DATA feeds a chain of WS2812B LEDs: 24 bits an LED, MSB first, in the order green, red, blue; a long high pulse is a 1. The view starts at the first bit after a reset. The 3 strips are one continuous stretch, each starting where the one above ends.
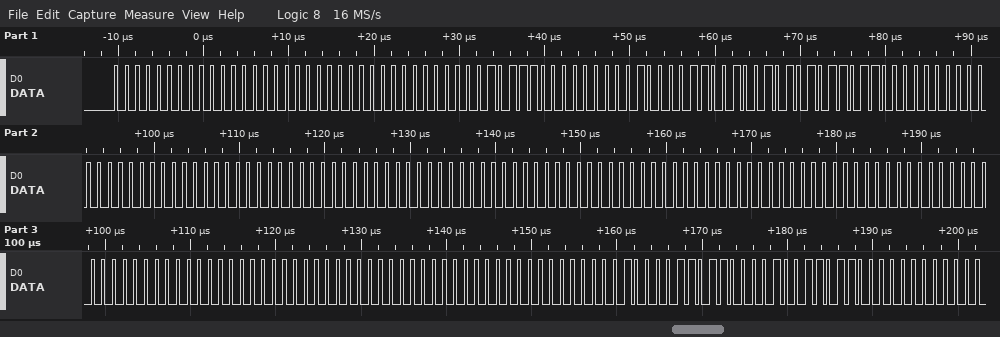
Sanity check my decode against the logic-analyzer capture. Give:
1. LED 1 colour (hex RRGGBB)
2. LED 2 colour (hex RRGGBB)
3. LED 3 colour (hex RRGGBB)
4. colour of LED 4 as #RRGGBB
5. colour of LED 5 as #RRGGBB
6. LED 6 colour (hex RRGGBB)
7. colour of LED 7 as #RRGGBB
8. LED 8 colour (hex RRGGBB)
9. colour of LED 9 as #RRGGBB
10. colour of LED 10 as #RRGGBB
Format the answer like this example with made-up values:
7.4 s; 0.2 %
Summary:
#000000; #170000; #25435B; #000000; #000000; #000000; #000000; #000000; #000000; #614336
